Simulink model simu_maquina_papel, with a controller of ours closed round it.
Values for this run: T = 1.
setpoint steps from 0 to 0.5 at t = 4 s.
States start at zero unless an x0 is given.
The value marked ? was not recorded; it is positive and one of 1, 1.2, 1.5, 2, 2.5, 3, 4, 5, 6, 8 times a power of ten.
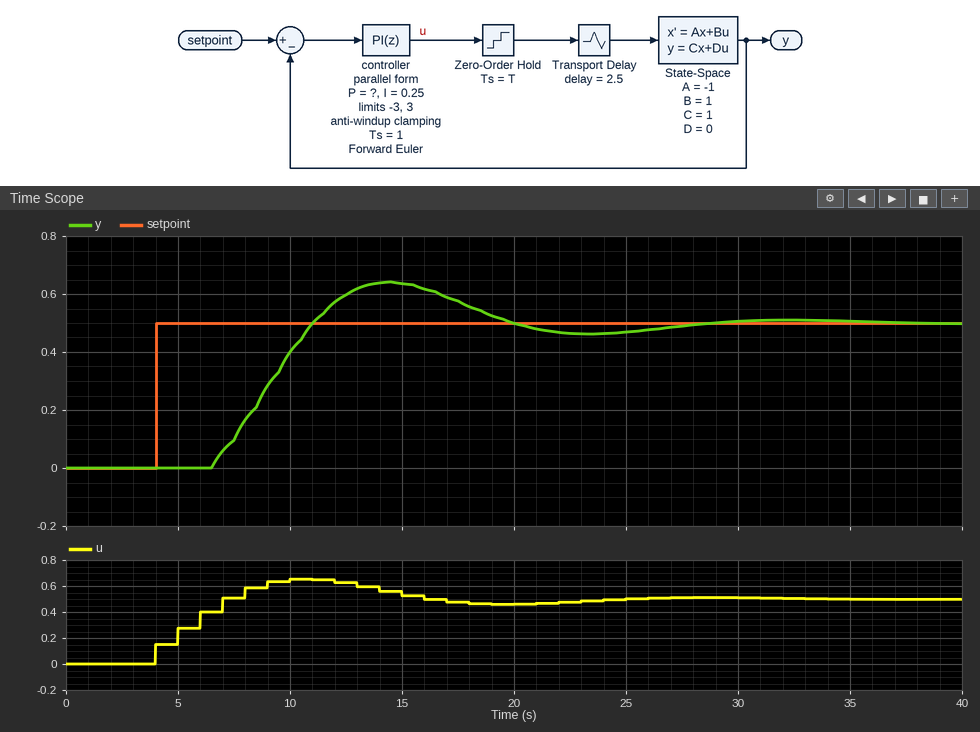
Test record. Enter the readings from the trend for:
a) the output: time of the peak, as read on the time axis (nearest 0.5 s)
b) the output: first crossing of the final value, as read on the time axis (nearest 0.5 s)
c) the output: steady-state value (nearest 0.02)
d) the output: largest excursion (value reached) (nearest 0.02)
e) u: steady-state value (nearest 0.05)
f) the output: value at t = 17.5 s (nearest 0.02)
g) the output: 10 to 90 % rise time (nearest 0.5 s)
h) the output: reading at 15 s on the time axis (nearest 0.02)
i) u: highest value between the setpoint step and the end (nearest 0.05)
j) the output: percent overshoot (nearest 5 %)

14.5 s
11.0 s
0.50
0.64
0.50
0.58
3.5 s
0.64
0.65
30 %
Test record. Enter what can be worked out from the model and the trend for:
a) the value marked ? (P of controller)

0.3
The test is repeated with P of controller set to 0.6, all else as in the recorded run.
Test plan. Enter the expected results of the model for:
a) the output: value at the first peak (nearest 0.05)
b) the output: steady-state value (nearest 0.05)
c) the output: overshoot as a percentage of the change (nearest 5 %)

0.60
0.50
15 %
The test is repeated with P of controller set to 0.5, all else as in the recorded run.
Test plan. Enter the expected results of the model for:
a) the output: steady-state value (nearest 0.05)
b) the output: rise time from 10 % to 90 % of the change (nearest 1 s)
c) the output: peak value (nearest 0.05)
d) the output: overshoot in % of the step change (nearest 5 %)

0.50
3 s
0.60
20 %
